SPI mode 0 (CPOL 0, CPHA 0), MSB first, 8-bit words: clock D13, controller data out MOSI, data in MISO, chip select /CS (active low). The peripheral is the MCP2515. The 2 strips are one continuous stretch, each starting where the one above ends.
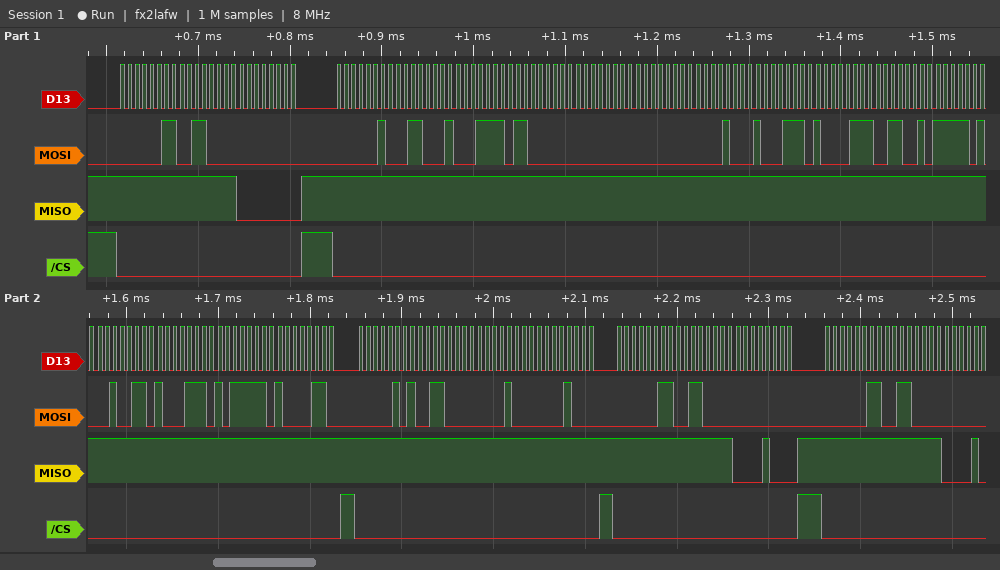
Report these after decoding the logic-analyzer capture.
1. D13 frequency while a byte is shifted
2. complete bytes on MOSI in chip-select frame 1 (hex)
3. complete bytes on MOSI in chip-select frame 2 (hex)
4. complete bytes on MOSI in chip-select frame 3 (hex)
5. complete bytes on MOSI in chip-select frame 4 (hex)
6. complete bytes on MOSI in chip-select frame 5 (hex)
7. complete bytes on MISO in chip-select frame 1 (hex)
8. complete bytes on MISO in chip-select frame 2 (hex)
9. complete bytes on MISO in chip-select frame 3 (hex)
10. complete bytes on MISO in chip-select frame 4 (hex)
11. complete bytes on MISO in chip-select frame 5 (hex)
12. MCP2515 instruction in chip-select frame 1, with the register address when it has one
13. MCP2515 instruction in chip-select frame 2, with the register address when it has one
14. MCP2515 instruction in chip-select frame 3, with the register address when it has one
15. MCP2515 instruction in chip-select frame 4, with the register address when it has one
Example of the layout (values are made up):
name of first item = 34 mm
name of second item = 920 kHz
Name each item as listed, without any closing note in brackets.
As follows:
D13 frequency while a byte is shifted = 125 kHz
complete bytes on MOSI in chip-select frame 1 = 03 30 00
complete bytes on MOSI in chip-select frame 2 = 02 31 1E C0 00 00 08 8E 87 32 FA 26 8E BE 86
complete bytes on MOSI in chip-select frame 3 = 05 30 08 08
complete bytes on MOSI in chip-select frame 4 = 03 30 00
complete bytes on MOSI in chip-select frame 5 = 03 30
complete bytes on MISO in chip-select frame 1 = FF FF 00
complete bytes on MISO in chip-select frame 2 = FF FF FF FF FF FF FF FF FF FF FF FF FF FF FF
complete bytes on MISO in chip-select frame 3 = FF FF FF FF
complete bytes on MISO in chip-select frame 4 = FF FF 08
complete bytes on MISO in chip-select frame 5 = FF FF
MCP2515 instruction in chip-select frame 1, with the register address when it has one = READ 0x30
MCP2515 instruction in chip-select frame 2, with the register address when it has one = WRITE 0x31
MCP2515 instruction in chip-select frame 3, with the register address when it has one = BIT MODIFY 0x30
MCP2515 instruction in chip-select frame 4, with the register address when it has one = READ 0x30
